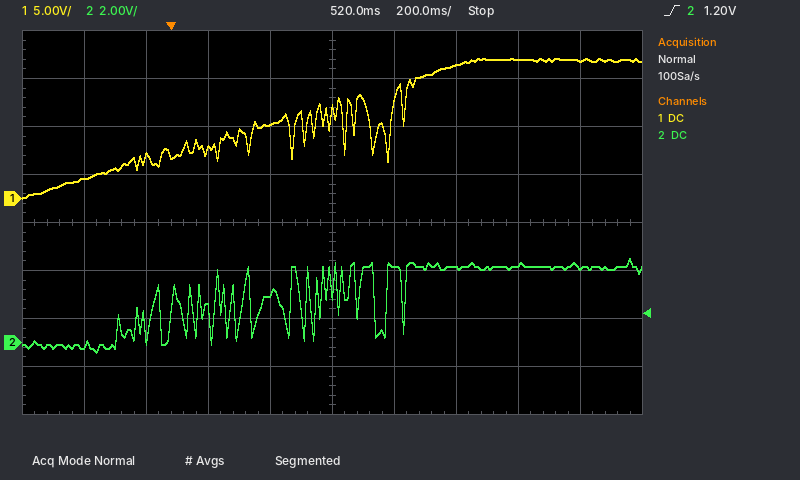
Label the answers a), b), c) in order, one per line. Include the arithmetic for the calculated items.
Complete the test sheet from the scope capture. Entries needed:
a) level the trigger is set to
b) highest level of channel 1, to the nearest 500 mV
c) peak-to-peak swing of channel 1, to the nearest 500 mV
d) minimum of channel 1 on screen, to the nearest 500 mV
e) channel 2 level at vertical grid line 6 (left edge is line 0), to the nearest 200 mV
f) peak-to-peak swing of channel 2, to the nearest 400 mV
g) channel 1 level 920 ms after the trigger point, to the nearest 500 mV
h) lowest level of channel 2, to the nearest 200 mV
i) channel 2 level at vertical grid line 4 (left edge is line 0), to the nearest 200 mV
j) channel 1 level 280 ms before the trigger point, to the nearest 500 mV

a) 1.20 V
b) 14.5 V
c) 14.5 V − (0.0 V) = 14.5 V
d) 0.0 V
e) 3.2 V
f) 4.0 V
g) 14.0 V
h) -400 mV
i) 2.0 V
j) 2.0 V
